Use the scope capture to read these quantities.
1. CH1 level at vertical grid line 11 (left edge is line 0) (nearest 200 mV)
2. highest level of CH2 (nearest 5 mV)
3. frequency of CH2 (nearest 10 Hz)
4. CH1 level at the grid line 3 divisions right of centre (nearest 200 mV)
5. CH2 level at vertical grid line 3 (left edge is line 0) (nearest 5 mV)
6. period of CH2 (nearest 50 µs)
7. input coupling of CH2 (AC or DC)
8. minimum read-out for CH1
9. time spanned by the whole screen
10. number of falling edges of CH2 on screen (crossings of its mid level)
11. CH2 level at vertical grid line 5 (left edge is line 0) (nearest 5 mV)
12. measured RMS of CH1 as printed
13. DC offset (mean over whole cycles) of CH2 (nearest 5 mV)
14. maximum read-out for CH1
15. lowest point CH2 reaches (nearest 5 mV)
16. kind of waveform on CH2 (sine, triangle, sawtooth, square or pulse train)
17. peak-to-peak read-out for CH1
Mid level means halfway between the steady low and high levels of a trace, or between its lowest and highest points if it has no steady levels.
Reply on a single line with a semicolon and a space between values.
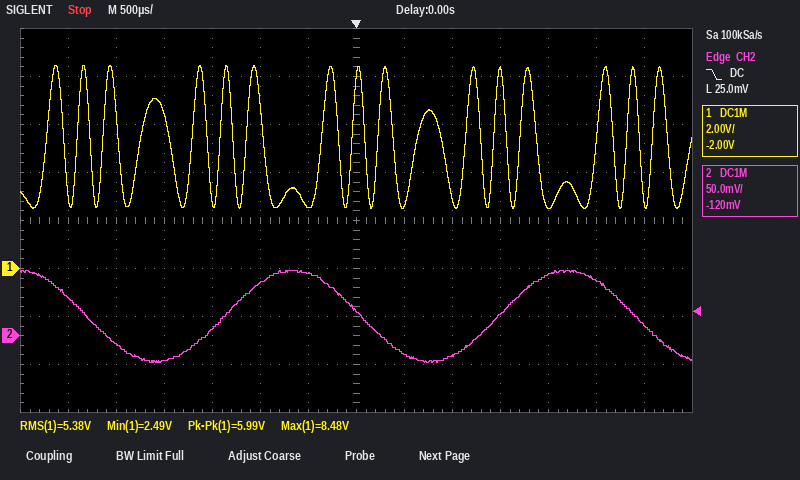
2.6 V; 70 mV; 350 Hz; 8.2 V; -25 mV; 2.85 ms; DC; 2.49 V; 7 ms; 3; 55 mV; 5.38 V; 20 mV; 8.48 V; -30 mV; sine; 5.99 V
